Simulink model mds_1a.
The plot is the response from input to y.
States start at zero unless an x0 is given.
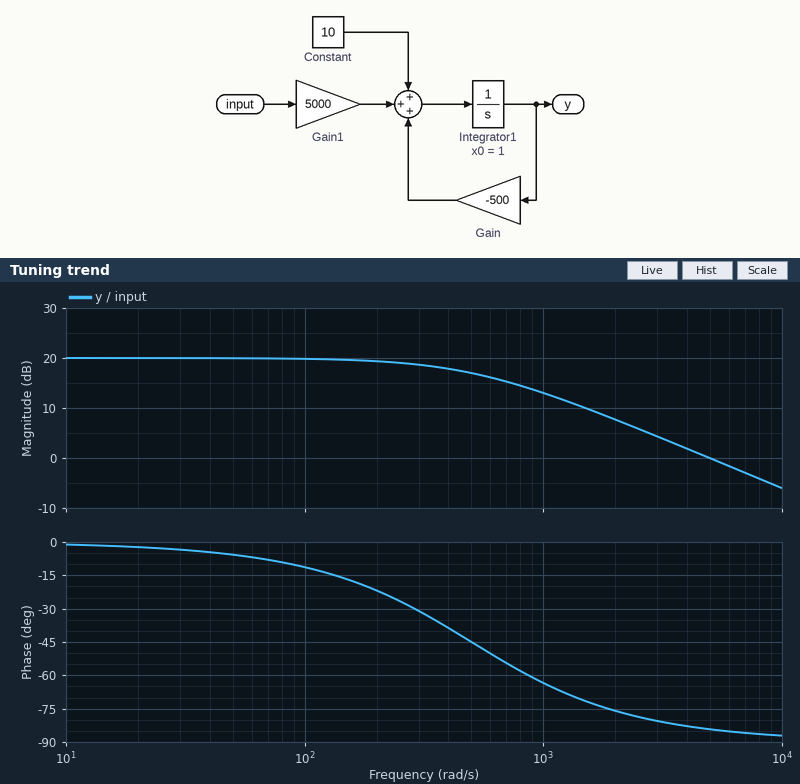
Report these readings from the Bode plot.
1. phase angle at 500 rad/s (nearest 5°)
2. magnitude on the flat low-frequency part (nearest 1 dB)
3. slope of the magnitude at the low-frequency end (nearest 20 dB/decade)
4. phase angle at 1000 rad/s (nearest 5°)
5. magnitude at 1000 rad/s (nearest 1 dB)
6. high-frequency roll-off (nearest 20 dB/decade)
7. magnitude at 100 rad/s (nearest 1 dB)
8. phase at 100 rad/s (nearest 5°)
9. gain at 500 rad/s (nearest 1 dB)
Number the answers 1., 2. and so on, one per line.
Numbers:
1. -45°
2. 20 dB
3. 0 dB/decade
4. -65°
5. 13 dB
6. -20 dB/decade
7. 20 dB
8. -10°
9. 17 dB
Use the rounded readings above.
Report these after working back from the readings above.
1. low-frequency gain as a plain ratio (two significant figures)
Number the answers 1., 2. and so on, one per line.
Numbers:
1. 10
